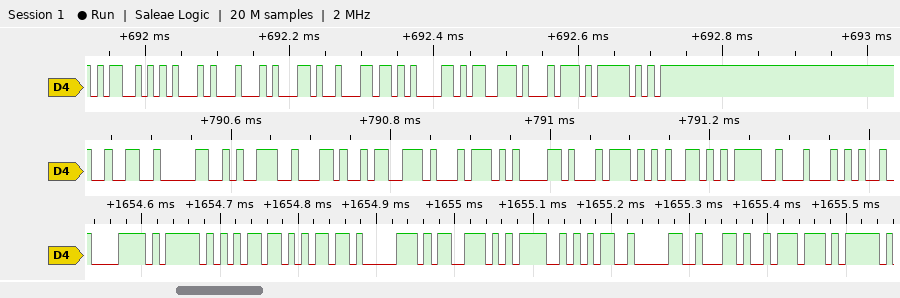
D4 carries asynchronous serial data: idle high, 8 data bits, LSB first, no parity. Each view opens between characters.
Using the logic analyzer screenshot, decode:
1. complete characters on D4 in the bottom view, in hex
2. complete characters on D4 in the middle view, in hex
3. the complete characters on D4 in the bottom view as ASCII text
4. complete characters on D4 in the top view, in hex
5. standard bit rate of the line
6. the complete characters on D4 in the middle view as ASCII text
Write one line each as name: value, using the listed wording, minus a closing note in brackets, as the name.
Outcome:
complete characters on D4 in the bottom view, in hex: 78, 5F, 6D, 6D, 70, 73, 3D, 35, 30, 2C, 77
complete characters on D4 in the middle view, in hex: 32, 30, 39, 2C, 73, 74, 61, 74, 65, 3D, 44
the complete characters on D4 in the bottom view as ASCII text: "x_mmps=50,w"
complete characters on D4 in the top view, in hex: 4D, 45, 44, 2C, 6C, 61, 73, 74, 5F, FF
standard bit rate of the line: 115200 baud
the complete characters on D4 in the middle view as ASCII text: "209,state=D"
